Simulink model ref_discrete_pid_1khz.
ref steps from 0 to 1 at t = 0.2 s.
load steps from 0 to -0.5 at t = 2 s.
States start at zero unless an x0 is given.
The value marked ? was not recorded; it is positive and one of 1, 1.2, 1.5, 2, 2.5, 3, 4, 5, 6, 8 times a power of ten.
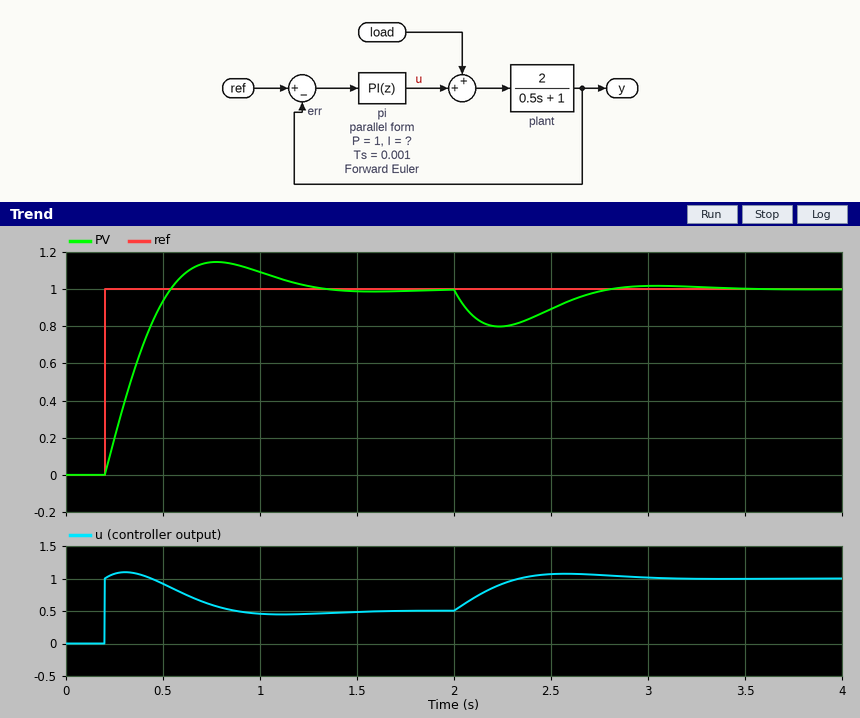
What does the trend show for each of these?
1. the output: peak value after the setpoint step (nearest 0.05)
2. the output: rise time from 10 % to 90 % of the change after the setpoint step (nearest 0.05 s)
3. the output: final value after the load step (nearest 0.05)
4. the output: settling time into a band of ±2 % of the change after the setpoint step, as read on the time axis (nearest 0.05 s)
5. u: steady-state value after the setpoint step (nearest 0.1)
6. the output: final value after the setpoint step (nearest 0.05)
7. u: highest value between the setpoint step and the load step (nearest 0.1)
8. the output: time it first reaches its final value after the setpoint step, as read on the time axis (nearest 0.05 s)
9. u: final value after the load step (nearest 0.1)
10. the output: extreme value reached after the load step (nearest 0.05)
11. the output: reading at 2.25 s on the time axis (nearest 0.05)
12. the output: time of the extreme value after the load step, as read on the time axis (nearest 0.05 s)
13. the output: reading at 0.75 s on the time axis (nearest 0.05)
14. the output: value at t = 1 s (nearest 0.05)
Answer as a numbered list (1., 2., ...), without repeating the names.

1. 1.15
2. 0.25 s
3. 1.00
4. 1.25 s
5. 0.5
6. 1.00
7. 1.1
8. 0.55 s
9. 1.0
10. 0.80
11. 0.80
12. 2.25 s
13. 1.15
14. 1.10
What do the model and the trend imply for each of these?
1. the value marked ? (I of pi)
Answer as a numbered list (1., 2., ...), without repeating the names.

1. 6
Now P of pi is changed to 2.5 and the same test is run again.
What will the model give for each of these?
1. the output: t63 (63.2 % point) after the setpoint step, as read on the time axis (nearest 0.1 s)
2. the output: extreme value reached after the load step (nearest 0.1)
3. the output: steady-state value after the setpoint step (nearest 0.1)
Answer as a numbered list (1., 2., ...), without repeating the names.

1. 0.3 s
2. 0.9
3. 1.0
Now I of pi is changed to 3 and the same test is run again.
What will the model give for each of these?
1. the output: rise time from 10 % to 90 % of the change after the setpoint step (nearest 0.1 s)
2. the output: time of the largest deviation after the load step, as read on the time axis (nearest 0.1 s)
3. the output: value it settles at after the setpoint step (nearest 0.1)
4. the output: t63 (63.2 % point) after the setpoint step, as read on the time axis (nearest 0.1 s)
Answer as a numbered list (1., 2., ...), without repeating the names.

1. 0.4 s
2. 2.3 s
3. 1.0
4. 0.4 s
